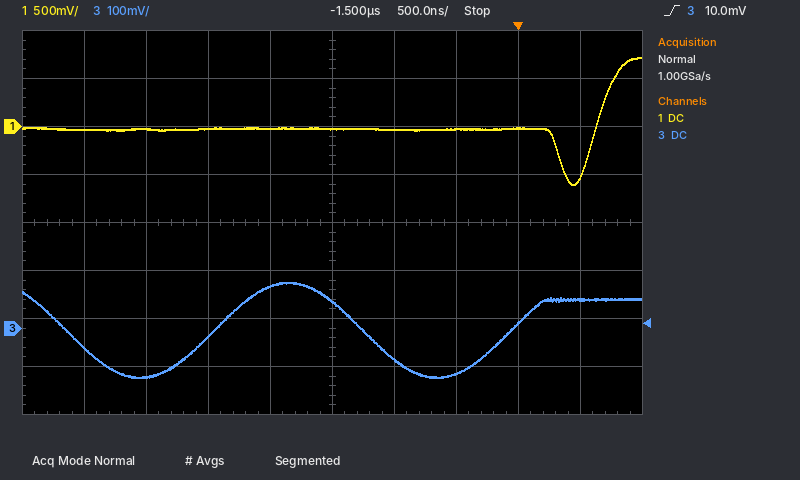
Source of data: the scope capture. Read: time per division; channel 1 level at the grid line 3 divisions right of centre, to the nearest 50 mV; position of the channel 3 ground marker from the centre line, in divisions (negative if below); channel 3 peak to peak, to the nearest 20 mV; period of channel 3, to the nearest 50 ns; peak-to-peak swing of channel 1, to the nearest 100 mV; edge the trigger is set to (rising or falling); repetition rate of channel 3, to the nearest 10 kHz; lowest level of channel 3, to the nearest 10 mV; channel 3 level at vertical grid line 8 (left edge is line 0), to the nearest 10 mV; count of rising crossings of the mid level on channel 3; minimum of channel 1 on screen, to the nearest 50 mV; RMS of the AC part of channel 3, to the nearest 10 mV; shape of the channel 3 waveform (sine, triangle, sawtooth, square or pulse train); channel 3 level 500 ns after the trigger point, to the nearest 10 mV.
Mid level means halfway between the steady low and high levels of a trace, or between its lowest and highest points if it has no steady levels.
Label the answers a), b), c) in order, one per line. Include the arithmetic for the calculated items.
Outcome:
a) 500 ns
b) 0 mV
c) -2.2 div
d) 200 mV
e) 2.40 µs
f) 1.30 V
g) rising
h) 1 / 2.40 µs ≈ 417 kHz, so 420 kHz to the nearest 10 kHz
i) -100 mV
j) 10 mV
k) 2
l) -600 mV
m) 200 mV / (2√2) ≈ 70.7 mV, so 70 mV to the nearest 10 mV
n) sine
o) 60 mV
